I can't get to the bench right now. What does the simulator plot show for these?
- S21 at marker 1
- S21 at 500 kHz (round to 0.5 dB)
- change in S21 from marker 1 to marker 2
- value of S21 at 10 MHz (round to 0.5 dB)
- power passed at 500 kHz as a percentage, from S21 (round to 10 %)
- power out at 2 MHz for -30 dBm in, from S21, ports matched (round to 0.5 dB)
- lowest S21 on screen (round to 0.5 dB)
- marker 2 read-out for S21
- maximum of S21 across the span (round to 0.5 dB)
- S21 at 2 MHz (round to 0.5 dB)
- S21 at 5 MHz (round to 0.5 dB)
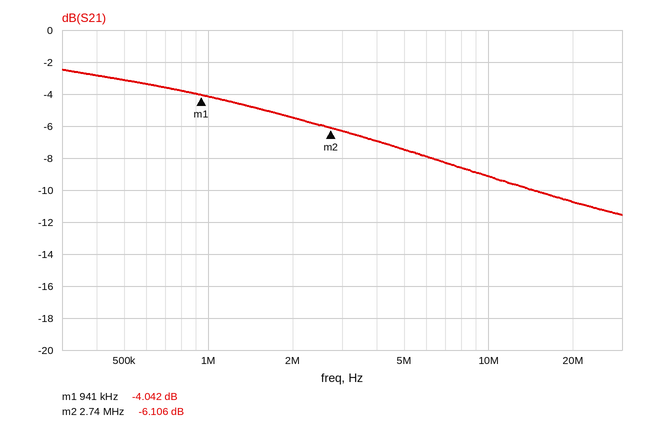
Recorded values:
-4.042 dB
-3.0 dB
-2.064 dB
-9.0 dB
50 %
-35.5 dBm
-11.5 dB
-6.106 dB
-2.5 dB
-5.5 dB
-7.5 dB
